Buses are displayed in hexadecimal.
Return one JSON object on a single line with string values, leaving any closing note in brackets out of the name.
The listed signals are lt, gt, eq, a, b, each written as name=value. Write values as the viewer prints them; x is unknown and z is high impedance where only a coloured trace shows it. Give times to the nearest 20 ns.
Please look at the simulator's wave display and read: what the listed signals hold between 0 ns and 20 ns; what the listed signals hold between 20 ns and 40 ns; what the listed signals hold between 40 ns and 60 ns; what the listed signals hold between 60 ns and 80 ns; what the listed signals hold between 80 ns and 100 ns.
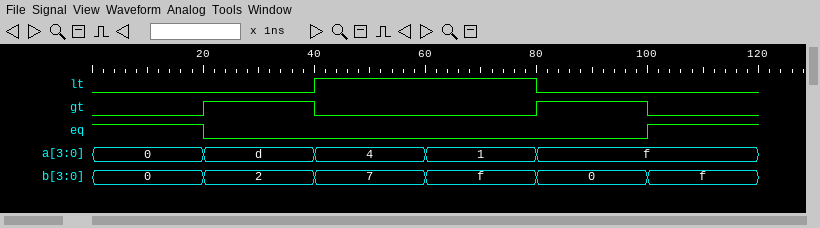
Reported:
{"what the listed signals hold between 0 ns and 20 ns": "lt=0, gt=0, eq=1, a=0, b=0", "what the listed signals hold between 20 ns and 40 ns": "lt=0, gt=1, eq=0, a=d, b=2", "what the listed signals hold between 40 ns and 60 ns": "lt=1, gt=0, eq=0, a=4, b=7", "what the listed signals hold between 60 ns and 80 ns": "lt=1, gt=0, eq=0, a=1, b=f", "what the listed signals hold between 80 ns and 100 ns": "lt=0, gt=1, eq=0, a=f, b=0"}
